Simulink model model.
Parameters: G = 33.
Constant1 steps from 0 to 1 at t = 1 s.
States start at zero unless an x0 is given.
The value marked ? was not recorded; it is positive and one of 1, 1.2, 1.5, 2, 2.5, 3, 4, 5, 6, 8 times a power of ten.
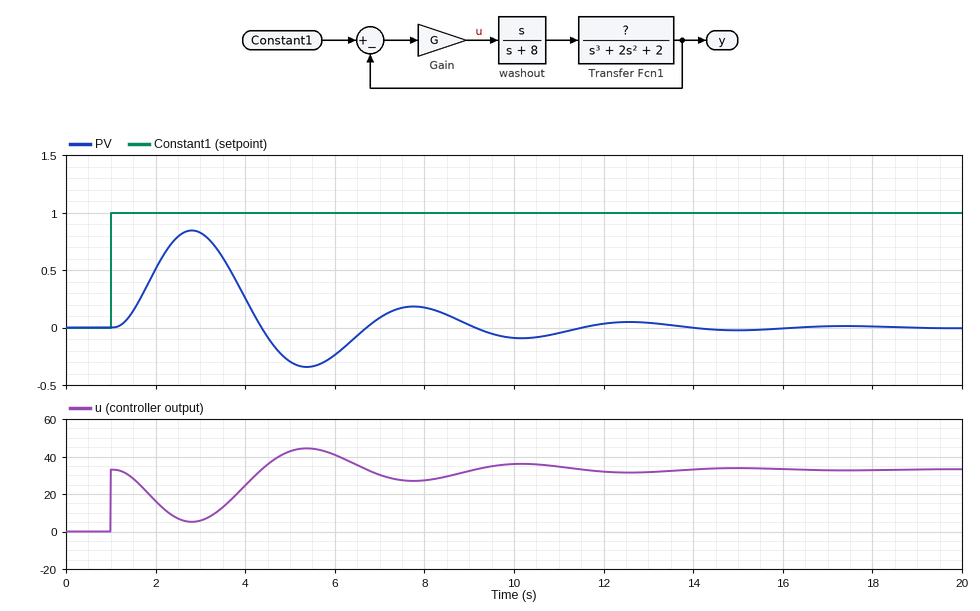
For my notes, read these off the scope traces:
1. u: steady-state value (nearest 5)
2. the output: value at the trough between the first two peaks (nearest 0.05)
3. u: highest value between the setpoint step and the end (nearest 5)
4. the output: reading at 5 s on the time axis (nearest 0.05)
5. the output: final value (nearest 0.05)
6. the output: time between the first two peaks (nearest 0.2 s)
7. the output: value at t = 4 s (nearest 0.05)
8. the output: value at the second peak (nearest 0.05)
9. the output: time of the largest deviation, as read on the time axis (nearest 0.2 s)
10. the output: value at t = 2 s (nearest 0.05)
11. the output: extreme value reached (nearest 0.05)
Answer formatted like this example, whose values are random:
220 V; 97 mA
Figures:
35; -0.35; 45; -0.30; 0.00; 5.0 s; 0.25; 0.20; 2.8 s; 0.50; 0.85
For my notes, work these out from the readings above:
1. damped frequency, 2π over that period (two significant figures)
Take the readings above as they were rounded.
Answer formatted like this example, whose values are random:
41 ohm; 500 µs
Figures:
1.3 rad/s
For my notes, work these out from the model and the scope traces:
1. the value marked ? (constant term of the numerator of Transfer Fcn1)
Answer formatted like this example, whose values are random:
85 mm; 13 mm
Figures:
0.6
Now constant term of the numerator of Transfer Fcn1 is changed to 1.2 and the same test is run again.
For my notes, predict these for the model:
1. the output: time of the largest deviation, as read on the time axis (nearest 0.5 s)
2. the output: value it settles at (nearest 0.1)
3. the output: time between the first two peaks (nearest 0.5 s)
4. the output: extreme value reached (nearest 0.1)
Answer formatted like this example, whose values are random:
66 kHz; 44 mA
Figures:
2.5 s; 0.0; 3.0 s; 1.2
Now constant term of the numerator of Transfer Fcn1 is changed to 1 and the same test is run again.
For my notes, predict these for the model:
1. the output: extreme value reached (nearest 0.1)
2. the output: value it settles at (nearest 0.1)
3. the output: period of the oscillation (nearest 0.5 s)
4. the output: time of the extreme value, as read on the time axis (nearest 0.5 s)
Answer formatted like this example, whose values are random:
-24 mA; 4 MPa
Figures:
1.1; 0.0; 3.5 s; 2.5 s
